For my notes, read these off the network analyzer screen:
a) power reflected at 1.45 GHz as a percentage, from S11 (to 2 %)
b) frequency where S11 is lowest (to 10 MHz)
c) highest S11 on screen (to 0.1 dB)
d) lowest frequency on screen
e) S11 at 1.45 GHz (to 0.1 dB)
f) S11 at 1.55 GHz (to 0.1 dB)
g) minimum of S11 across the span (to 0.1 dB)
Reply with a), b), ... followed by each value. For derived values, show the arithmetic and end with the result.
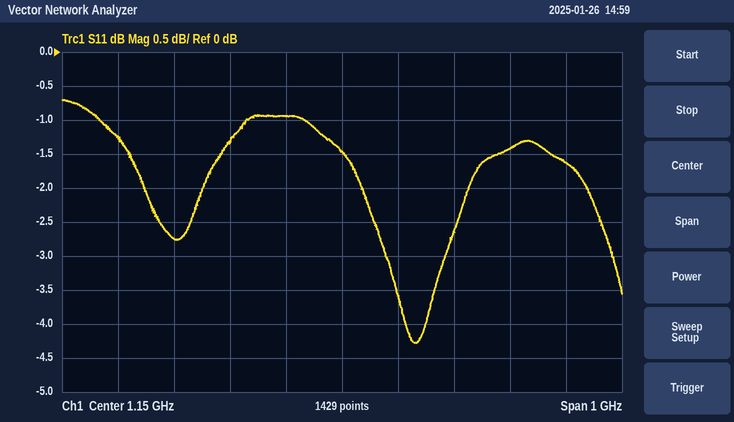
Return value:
a) 10^(-1.4/10) ≈ 72 %
b) 1.28 GHz
c) -0.7 dB
d) 650 MHz
e) -1.4 dB
f) -1.6 dB
g) -4.3 dB
